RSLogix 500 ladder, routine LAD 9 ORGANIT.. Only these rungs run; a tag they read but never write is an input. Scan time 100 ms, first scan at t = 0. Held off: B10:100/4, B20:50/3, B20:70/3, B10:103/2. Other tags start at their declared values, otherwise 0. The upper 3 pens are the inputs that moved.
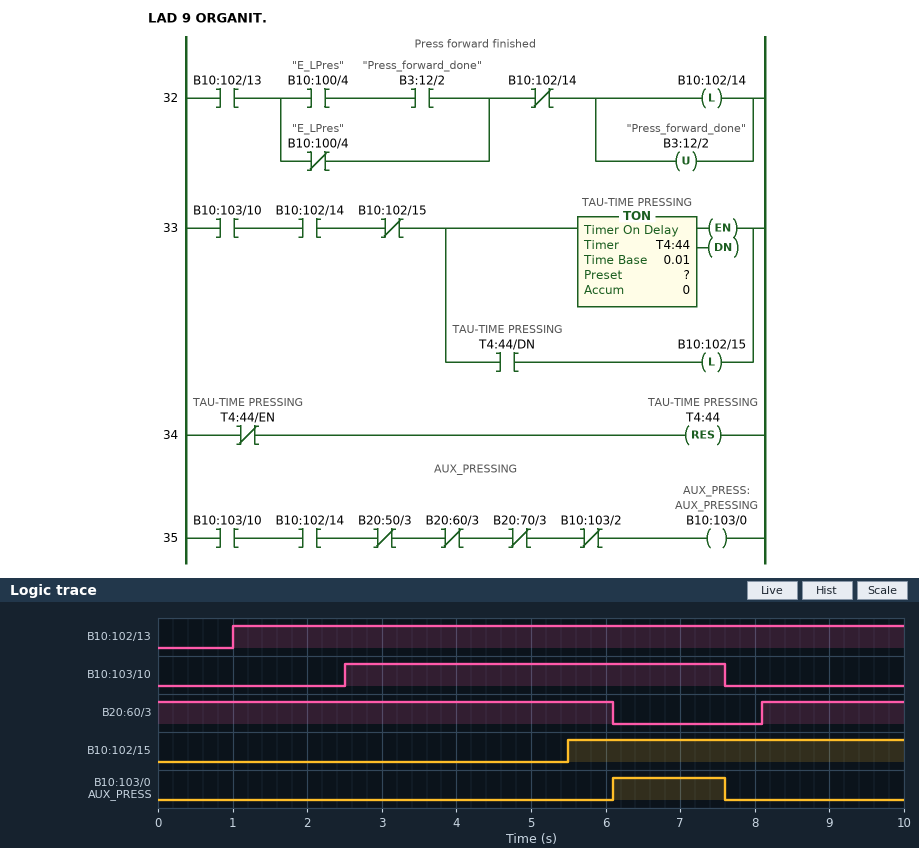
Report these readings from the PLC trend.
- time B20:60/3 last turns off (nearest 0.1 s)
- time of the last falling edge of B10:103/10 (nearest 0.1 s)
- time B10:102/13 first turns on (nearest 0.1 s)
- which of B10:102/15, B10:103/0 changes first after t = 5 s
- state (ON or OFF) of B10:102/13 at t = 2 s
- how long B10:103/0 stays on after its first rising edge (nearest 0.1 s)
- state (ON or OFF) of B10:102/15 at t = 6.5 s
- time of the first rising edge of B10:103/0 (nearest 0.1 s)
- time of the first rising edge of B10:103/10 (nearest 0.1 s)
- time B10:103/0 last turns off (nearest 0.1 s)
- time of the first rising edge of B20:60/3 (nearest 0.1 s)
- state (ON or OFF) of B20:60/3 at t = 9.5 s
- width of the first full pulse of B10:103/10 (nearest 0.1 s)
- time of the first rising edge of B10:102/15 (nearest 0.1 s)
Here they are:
6.1 s
7.6 s
1.0 s
B10:102/15
ON
1.5 s
ON
6.1 s
2.5 s
7.6 s
8.1 s
ON
5.1 s
5.5 s
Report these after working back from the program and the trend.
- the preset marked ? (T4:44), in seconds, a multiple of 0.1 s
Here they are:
3.0 s
